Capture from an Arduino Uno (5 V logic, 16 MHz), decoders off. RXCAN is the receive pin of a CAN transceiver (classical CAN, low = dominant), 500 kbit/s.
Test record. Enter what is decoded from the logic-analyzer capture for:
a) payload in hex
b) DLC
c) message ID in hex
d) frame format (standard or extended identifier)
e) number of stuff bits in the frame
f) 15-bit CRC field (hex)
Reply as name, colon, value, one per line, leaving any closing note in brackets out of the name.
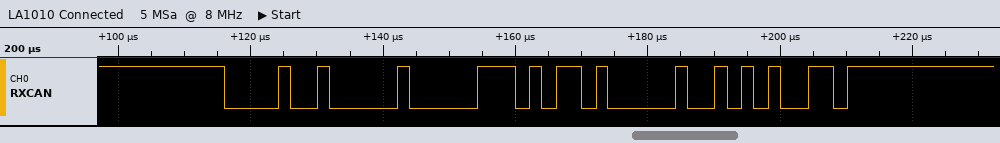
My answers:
payload in hex: AD
DLC: 1
message ID in hex: 0x090
frame format: standard
number of stuff bits in the frame: 3
15-bit CRC field: 0x00A9
